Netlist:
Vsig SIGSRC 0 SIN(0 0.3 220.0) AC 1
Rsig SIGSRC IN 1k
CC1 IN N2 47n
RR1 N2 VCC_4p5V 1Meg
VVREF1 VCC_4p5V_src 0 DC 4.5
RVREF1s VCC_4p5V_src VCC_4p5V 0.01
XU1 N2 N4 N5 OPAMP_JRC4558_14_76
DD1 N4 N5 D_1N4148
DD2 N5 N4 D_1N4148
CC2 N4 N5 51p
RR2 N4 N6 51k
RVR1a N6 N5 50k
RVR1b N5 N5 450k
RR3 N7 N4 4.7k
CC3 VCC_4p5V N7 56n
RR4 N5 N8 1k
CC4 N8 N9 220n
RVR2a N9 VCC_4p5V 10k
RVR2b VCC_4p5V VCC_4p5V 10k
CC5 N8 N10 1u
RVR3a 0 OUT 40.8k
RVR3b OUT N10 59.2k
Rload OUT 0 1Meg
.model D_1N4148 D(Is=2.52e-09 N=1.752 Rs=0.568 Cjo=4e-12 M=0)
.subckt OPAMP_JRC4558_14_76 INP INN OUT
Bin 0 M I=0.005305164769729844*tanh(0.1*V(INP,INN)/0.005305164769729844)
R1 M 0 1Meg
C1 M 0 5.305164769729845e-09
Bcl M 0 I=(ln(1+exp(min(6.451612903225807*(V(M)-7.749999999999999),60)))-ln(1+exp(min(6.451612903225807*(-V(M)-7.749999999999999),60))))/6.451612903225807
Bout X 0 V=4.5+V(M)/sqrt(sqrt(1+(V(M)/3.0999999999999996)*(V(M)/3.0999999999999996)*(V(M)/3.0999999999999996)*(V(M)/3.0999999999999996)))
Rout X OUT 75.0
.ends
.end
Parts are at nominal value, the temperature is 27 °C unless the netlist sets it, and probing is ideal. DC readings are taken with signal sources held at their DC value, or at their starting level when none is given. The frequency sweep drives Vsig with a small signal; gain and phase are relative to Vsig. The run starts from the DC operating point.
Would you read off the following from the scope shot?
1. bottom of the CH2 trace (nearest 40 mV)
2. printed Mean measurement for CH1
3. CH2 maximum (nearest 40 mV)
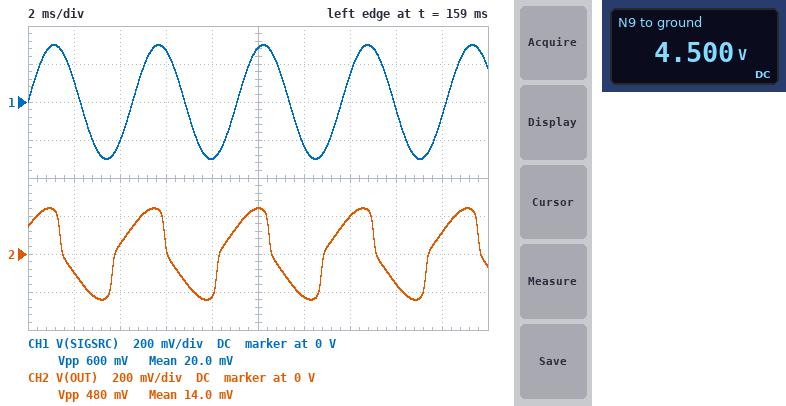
-240 mV
20.0 mV
240 mV
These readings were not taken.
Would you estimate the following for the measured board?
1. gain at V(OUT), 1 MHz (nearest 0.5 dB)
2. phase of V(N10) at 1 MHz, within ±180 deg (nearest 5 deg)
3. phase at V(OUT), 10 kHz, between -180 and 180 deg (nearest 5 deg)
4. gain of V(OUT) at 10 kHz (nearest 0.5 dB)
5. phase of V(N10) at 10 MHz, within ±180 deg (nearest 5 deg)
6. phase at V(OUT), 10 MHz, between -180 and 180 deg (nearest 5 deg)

-9.5 dB
-45 deg
-20 deg
17.5 dB
-75 deg
-75 deg
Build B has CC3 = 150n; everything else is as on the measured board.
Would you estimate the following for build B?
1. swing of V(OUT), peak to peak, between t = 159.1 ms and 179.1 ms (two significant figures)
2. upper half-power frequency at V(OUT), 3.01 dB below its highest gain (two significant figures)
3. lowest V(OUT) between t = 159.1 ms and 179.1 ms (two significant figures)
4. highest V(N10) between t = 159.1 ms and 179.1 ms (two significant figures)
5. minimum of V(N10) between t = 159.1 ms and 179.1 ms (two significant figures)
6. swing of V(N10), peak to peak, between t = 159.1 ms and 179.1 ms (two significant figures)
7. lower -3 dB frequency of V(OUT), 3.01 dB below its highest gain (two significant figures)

530 mV
23 kHz
-260 mV
660 mV
-660 mV
1.3 V
220 Hz
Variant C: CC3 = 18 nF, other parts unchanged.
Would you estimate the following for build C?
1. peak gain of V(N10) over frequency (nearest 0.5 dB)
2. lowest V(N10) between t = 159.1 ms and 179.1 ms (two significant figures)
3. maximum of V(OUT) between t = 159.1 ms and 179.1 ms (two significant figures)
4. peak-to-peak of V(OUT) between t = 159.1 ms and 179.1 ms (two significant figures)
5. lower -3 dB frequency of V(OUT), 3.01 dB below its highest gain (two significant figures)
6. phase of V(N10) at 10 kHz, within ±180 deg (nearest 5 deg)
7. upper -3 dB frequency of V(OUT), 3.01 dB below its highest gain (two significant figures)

25.5 dB
-500 mV
200 mV
400 mV
1.6 kHz
-15 deg
26 kHz
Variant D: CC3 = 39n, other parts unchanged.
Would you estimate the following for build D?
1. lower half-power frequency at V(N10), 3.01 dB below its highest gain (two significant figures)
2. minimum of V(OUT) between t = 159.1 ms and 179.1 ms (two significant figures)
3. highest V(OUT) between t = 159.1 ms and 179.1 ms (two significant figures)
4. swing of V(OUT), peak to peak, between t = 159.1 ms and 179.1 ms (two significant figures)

810 Hz
-230 mV
230 mV
460 mV
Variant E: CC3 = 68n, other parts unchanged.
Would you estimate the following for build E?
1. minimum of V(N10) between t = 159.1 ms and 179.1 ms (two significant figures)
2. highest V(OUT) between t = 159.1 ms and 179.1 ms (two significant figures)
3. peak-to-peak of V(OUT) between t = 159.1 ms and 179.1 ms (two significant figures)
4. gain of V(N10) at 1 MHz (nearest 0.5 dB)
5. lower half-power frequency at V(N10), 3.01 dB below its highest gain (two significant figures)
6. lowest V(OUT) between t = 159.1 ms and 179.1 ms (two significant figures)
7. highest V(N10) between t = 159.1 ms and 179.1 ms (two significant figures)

-620 mV
250 mV
490 mV
-1.5 dB
480 Hz
-250 mV
620 mV
